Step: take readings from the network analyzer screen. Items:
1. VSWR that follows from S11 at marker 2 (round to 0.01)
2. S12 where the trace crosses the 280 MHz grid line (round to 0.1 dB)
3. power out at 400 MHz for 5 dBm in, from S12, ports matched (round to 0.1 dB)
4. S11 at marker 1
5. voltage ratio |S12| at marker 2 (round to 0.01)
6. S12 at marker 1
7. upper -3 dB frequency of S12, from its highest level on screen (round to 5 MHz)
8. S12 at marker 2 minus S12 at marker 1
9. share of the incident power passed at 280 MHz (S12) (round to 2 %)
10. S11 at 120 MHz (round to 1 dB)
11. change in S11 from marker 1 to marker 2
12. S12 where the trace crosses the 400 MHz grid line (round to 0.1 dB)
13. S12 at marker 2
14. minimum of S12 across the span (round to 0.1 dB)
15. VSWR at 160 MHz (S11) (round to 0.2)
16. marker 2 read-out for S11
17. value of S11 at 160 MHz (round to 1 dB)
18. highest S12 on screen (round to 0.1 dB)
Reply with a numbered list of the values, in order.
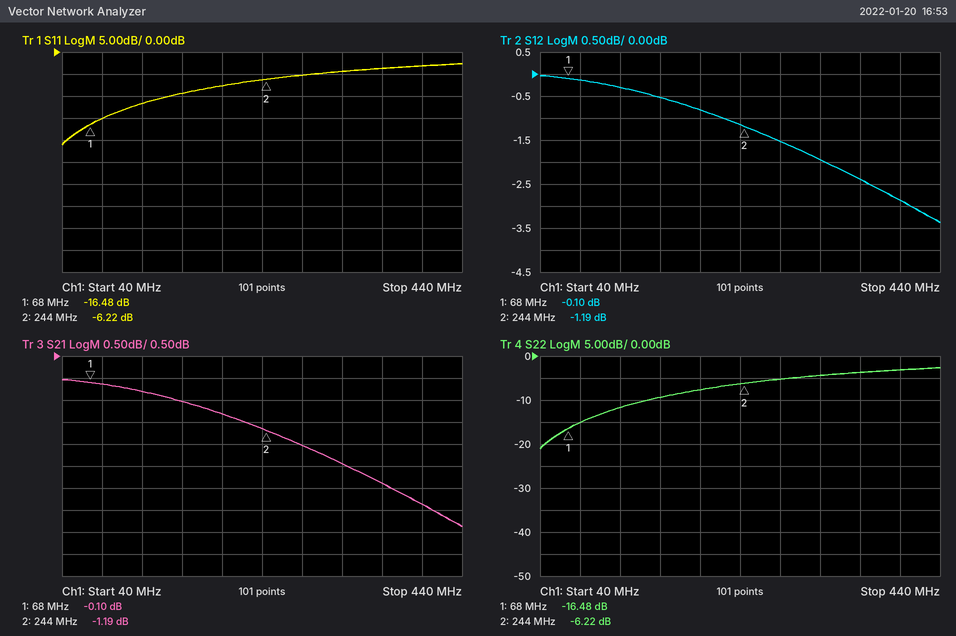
1. 2.91
2. -1.5 dB
3. 2.1 dBm
4. -16.48 dB
5. 0.87
6. -0.10 dB
7. 415 MHz
8. -1.09 dB
9. 70 %
10. -12 dB
11. 10.26 dB
12. -2.9 dB
13. -1.19 dB
14. -3.4 dB
15. 2.0
16. -6.22 dB
17. -9 dB
18. 0.0 dB
